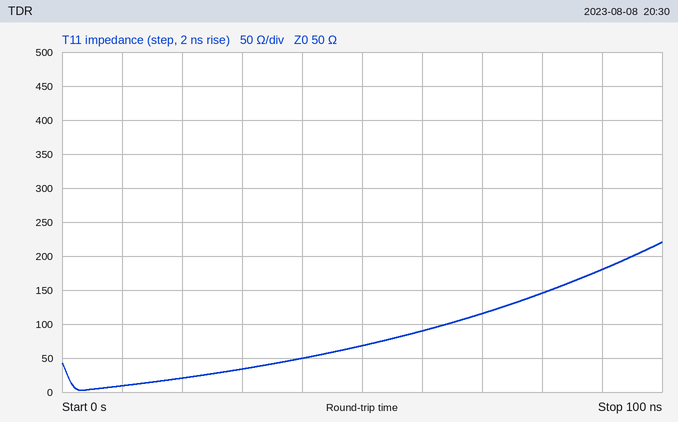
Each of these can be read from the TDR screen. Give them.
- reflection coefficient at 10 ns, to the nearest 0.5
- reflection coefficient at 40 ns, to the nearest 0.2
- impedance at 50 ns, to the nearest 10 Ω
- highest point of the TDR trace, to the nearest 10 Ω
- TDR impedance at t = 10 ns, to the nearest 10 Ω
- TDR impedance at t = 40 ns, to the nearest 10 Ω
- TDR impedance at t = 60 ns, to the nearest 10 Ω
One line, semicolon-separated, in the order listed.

-0.5; 0.0; 70 Ω; 220 Ω; 10 Ω; 50 Ω; 90 Ω
